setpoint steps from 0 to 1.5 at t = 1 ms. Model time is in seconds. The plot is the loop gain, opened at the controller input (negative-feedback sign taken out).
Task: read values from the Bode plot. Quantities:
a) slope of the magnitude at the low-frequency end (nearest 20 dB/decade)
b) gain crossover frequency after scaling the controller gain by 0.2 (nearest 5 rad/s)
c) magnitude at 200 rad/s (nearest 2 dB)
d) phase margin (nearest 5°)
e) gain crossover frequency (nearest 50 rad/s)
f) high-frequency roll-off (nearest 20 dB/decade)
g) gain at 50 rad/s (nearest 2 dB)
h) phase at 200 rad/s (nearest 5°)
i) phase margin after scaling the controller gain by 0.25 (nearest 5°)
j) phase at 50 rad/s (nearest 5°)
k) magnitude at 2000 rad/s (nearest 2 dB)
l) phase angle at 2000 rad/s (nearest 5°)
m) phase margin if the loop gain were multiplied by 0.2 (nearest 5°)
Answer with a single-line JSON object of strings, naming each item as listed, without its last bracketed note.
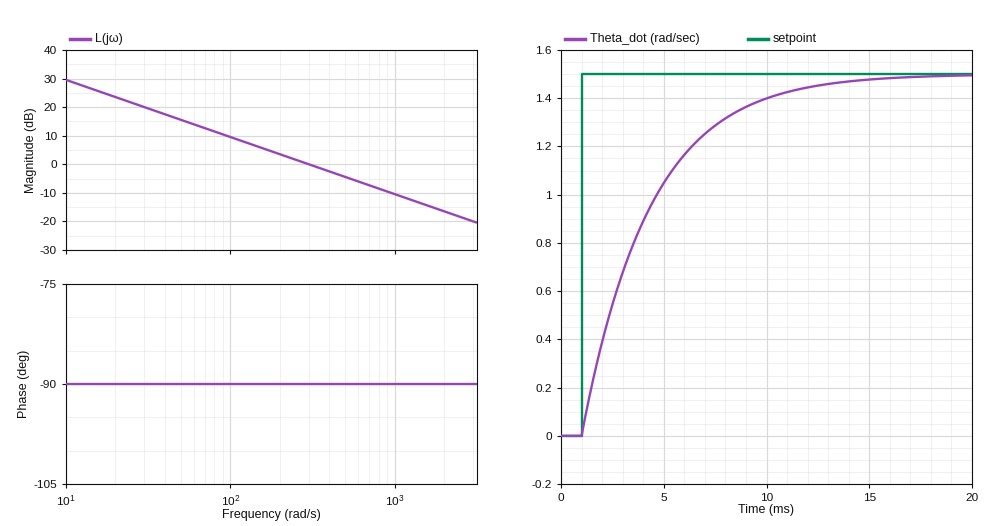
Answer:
{"slope of the magnitude at the low-frequency end": "-20 dB/decade", "gain crossover frequency after scaling the controller gain by 0.2": "60 rad/s", "magnitude at 200 rad/s": "4 dB", "phase margin": "90°", "gain crossover frequency": "300 rad/s", "high-frequency roll-off": "-20 dB/decade", "gain at 50 rad/s": "16 dB", "phase at 200 rad/s": "-90°", "phase margin after scaling the controller gain by 0.25": "90°", "phase at 50 rad/s": "-90°", "magnitude at 2000 rad/s": "-16 dB", "phase angle at 2000 rad/s": "-90°", "phase margin if the loop gain were multiplied by 0.2": "90°"}
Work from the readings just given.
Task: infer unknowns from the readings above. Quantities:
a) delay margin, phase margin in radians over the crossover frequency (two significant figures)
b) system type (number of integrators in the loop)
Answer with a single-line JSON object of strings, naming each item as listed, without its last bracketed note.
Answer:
{"delay margin, phase margin in radians over the crossover frequency": "0.0052 s", "system type": "1"}
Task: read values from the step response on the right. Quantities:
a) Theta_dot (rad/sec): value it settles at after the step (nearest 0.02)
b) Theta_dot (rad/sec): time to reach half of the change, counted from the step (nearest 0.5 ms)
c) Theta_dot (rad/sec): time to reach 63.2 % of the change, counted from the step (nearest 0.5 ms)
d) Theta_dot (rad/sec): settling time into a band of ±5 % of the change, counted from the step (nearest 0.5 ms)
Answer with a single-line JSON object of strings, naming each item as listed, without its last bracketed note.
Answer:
{"Theta_dot (rad/sec): value it settles at after the step": "1.50", "Theta_dot (rad/sec): time to reach half of the change, counted from the step": "2.5 ms", "Theta_dot (rad/sec): time to reach 63.2 % of the change, counted from the step": "3.5 ms", "Theta_dot (rad/sec): settling time into a band of ±5 % of the change, counted from the step": "10.0 ms"}
